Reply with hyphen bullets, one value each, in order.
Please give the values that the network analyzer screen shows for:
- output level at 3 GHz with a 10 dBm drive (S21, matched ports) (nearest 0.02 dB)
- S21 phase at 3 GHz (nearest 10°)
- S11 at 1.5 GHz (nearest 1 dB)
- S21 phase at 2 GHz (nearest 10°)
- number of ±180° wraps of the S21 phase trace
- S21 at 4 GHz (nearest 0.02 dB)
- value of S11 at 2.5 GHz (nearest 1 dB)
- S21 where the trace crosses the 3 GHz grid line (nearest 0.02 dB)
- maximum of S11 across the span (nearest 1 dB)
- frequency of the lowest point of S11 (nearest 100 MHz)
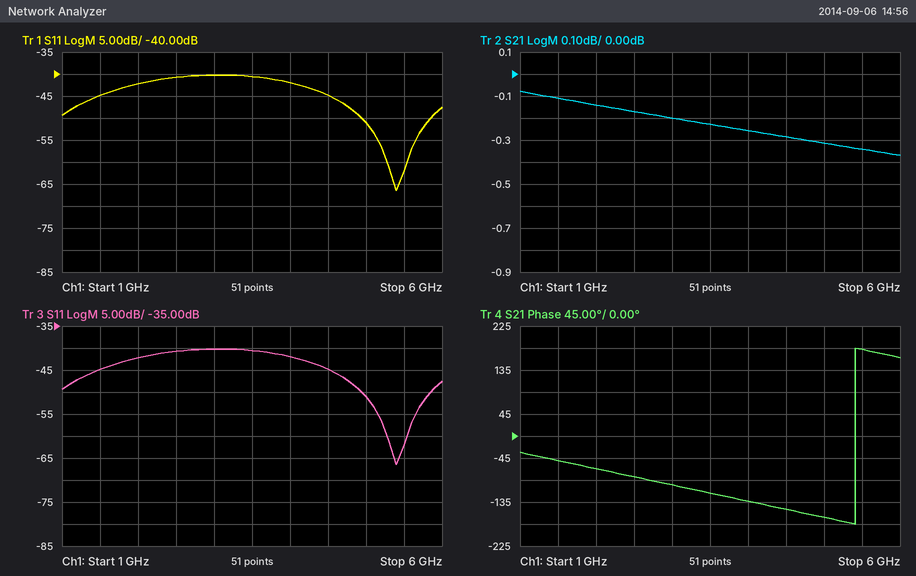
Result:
- 9.80 dBm
- -100°
- -45 dB
- -70°
- 1
- -0.26 dB
- -41 dB
- -0.20 dB
- -40 dB
- 5.4 GHz
